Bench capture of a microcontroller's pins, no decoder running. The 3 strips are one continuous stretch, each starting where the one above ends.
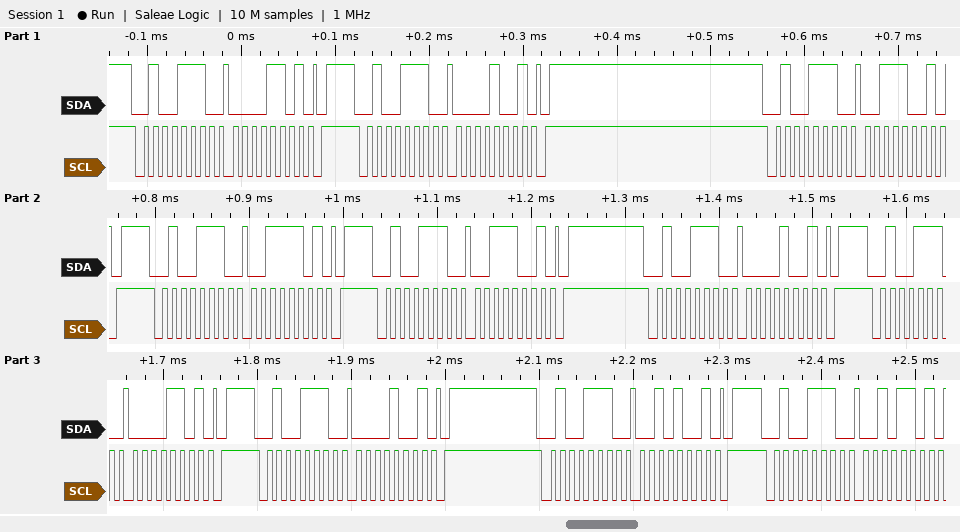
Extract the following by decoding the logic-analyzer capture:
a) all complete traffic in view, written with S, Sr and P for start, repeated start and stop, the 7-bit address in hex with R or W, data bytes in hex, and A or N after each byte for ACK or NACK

S 27W A 0D A P S 27W A 09 A P S 27W A 39 A P S 27W A 3D A P S 27W A 39 A P S 27W A 09 A P S 27W A 0D A P S 27W A 09 A P S 27W A 29 A P S 27W A 2D A
